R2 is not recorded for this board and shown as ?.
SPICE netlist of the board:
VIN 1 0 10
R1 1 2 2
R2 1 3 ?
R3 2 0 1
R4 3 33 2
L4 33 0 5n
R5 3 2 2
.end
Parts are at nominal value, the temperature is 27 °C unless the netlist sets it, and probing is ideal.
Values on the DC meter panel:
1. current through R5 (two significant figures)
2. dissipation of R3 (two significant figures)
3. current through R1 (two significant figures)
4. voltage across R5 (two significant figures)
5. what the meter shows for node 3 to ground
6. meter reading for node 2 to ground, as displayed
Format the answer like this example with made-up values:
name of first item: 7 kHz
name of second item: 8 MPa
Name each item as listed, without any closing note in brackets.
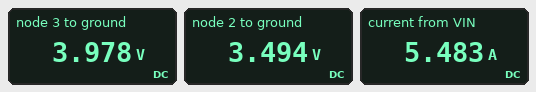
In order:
current through R5: 240 mA
dissipation of R3: 12 W
current through R1: 3.3 A
voltage across R5: 480 mV
what the meter shows for node 3 to ground: 3.978 V
meter reading for node 2 to ground, as displayed: 3.494 V
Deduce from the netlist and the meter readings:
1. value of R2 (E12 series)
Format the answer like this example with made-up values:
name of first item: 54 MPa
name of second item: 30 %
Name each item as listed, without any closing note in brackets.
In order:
value of R2: 2.7 Ω
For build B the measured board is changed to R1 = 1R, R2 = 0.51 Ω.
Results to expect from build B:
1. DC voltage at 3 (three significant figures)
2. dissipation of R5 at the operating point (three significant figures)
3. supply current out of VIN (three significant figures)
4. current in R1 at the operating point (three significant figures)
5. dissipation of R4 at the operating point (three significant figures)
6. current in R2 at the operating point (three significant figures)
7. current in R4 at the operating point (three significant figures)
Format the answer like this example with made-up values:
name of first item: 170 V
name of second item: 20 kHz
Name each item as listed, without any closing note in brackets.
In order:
DC voltage at 3: 7.55 V
dissipation of R5 at the operating point: 2.09 W
supply current out of VIN: 9.29 A
current in R1 at the operating point: 4.49 A
dissipation of R4 at the operating point: 28.5 W
current in R2 at the operating point: 4.80 A
current in R4 at the operating point: 3.78 A
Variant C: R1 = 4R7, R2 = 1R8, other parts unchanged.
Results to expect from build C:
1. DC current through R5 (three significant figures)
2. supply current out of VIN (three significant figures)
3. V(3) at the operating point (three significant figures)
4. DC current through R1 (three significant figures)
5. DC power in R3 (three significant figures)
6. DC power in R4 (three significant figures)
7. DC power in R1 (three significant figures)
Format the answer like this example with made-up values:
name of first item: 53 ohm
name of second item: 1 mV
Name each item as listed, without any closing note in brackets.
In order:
DC current through R5: 930 mA
supply current out of VIN: 4.71 A
V(3) at the operating point: 4.38 V
DC current through R1: 1.59 A
DC power in R3: 6.36 W
DC power in R4: 9.60 W
DC power in R1: 11.9 W
